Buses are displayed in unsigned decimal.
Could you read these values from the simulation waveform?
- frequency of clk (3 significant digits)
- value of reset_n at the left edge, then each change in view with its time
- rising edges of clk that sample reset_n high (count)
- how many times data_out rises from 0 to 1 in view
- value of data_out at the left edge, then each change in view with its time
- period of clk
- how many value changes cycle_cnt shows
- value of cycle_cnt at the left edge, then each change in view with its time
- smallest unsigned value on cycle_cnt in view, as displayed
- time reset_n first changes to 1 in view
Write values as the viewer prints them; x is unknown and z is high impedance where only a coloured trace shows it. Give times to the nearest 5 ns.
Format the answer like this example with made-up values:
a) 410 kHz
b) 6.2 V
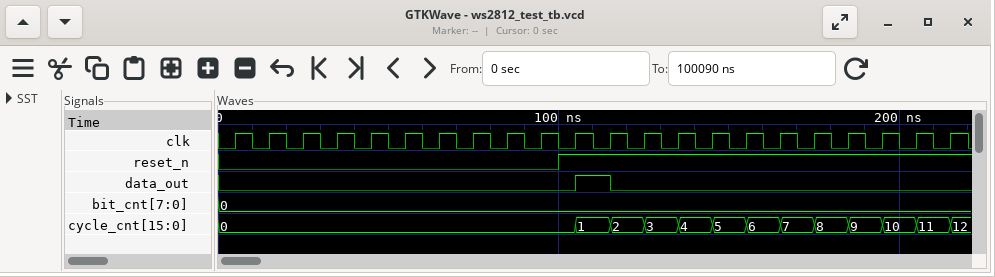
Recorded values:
a) 100 MHz
b) 0, 1 at 100 ns
c) 12
d) 1
e) 0, 1 at 105 ns, 0 at 115 ns
f) 10 ns
g) 12
h) 0, 1 at 105 ns, 2 at 115 ns, 3 at 125 ns, 4 at 135 ns, 5 at 145 ns, 6 at 155 ns, 7 at 165 ns, 8 at 175 ns, 9 at 185 ns, 10 at 195 ns, 11 at 205 ns, 12 at 215 ns
i) 0
j) 100 ns
